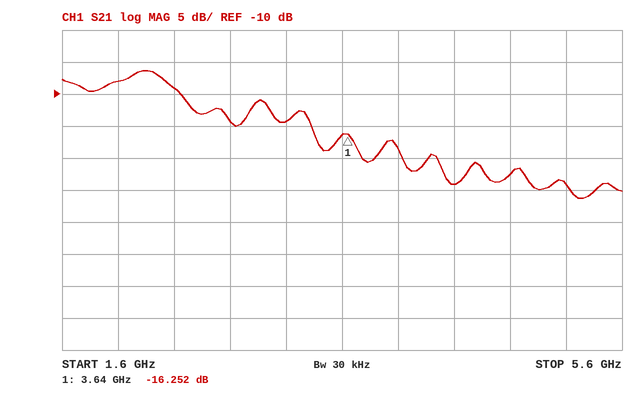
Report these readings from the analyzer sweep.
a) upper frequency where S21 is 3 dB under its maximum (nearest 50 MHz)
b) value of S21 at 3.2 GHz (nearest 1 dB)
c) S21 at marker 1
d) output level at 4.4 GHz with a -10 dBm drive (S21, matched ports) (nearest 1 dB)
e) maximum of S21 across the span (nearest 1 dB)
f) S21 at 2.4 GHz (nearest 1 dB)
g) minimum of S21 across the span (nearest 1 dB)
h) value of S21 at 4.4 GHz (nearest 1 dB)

2.40 GHz
-14 dB
-16.252 dB
-34 dBm
-6 dB
-9 dB
-26 dB
-24 dB
